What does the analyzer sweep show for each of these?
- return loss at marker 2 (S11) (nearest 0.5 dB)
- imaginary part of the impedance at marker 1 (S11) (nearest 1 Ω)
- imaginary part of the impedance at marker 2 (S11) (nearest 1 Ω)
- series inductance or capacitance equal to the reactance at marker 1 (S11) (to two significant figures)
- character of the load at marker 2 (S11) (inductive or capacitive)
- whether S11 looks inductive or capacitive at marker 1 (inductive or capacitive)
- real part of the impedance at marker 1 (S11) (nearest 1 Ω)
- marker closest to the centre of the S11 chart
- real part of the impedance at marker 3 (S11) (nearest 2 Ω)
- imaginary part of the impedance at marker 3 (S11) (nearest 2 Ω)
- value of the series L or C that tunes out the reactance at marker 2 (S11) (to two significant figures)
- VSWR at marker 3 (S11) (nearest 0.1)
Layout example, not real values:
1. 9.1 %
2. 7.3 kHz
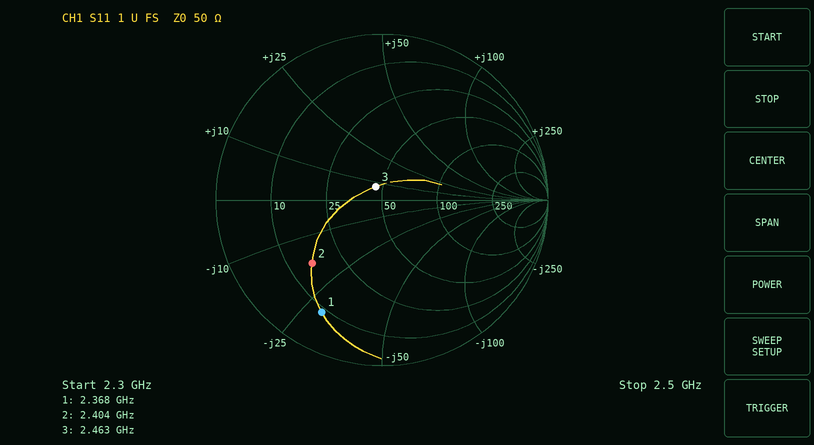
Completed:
1. 5.0 dB
2. -29 Ω
3. -18 Ω
4. 2.3 pF
5. capacitive
6. capacitive
7. 9 Ω
8. marker 3
9. 46 Ω
10. +8 Ω
11. 1.2 nH
12. 1.2
